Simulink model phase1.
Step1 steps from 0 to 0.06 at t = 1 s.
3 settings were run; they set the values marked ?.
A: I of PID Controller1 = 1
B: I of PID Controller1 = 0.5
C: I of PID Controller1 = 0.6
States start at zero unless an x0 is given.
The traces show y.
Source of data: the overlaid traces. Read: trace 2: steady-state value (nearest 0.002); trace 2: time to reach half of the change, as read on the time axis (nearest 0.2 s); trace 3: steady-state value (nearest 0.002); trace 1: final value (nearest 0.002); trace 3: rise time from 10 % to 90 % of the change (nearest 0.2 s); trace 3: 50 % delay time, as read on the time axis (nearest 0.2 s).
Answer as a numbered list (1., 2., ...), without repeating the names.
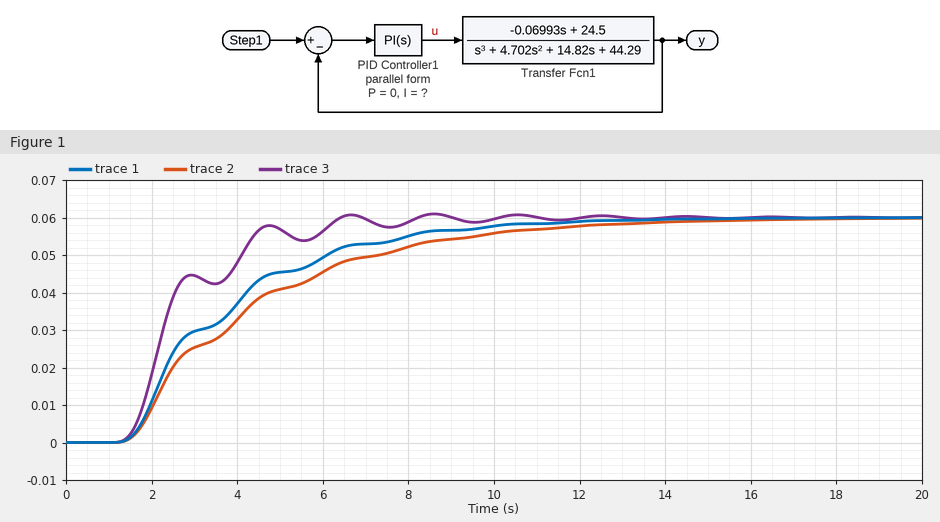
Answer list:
1. 0.060
2. 3.8 s
3. 0.060
4. 0.060
5. 2.6 s
6. 2.2 s
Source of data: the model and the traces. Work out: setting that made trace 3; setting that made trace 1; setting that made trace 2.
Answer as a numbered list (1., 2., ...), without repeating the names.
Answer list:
1. A
2. C
3. B
